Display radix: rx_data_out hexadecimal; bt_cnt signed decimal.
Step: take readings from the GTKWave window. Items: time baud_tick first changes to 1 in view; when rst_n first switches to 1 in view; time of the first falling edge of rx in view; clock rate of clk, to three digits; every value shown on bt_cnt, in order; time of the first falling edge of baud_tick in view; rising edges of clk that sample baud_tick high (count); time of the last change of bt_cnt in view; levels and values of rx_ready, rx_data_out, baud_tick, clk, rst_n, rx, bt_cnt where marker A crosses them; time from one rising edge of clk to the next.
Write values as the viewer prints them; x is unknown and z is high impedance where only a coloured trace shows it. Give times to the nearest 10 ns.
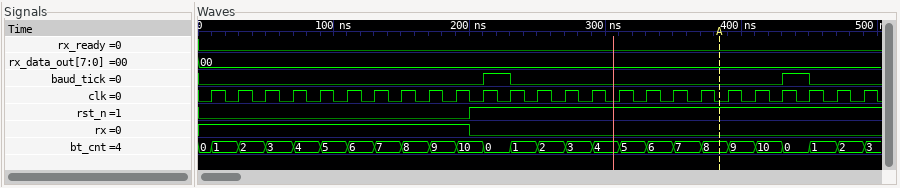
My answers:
210 ns
200 ns
200 ns
50.0 MHz
0, 1, 2, 3, 4, 5, 6, 7, 8, 9, 10, 0, 1, 2, 3, 4, 5, 6, 7, 8, 9, 10, 0, 1, 2, 3
230 ns
2
490 ns
rx_ready=0, rx_data_out=00, baud_tick=0, clk=0, rst_n=1, rx=0, bt_cnt=8
20 ns
